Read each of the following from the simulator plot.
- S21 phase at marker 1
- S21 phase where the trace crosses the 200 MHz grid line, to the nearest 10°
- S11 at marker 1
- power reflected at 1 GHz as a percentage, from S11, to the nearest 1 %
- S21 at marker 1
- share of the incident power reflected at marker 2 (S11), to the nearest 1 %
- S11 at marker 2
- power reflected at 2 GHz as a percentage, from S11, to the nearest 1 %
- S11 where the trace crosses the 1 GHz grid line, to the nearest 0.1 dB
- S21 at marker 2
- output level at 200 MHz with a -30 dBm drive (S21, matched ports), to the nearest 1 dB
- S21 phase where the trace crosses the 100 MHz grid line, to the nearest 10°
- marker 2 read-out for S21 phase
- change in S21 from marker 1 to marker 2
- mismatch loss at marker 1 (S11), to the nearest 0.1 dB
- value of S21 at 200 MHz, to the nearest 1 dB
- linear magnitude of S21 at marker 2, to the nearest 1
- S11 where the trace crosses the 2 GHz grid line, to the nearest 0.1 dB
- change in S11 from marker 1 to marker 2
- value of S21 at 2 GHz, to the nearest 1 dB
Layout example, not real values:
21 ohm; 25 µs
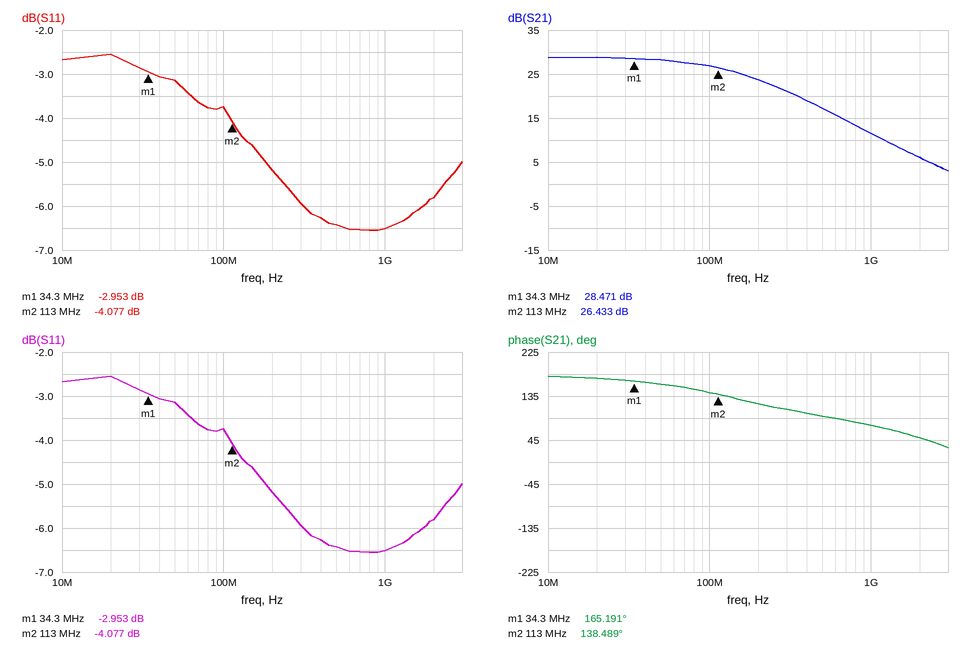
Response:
165.191°; 120°; -2.953 dB; 22 %; 28.471 dB; 39 %; -4.077 dB; 26 %; -6.5 dB; 26.433 dB; -6 dBm; 140°; 138.489°; -2.038 dB; 3.1 dB; 24 dB; 21; -5.8 dB; -1.124 dB; 6 dB
